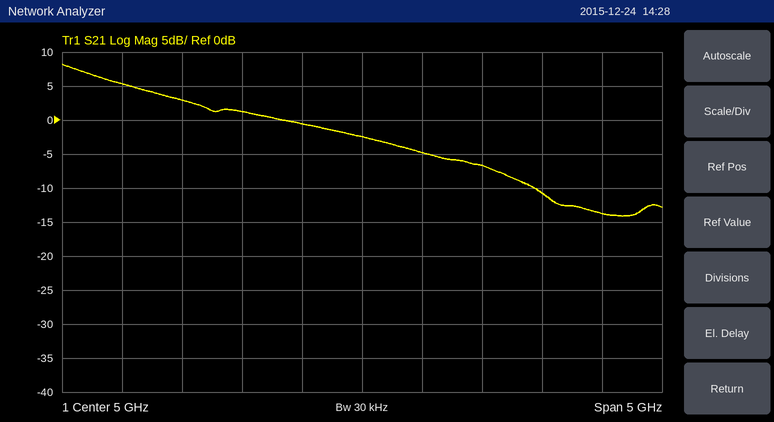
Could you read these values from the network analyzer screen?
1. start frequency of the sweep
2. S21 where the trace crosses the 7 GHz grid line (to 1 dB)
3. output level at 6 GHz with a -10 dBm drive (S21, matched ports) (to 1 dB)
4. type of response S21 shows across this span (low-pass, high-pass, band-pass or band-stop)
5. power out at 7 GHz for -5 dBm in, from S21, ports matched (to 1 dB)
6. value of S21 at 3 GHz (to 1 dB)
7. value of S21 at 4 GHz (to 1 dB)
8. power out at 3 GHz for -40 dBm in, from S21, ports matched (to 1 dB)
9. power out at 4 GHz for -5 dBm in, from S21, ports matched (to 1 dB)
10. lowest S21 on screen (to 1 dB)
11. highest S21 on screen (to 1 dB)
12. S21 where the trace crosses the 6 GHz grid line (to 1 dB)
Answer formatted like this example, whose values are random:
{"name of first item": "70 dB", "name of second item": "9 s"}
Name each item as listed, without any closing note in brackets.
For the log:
{"start frequency of the sweep": "2.5 GHz", "S21 where the trace crosses the 7 GHz grid line": "-14 dB", "output level at 6 GHz with a -10 dBm drive (S21, matched ports)": "-17 dBm", "type of response S21 shows across this span": "low-pass", "power out at 7 GHz for -5 dBm in, from S21, ports matched": "-19 dBm", "value of S21 at 3 GHz": "5 dB", "value of S21 at 4 GHz": "1 dB", "power out at 3 GHz for -40 dBm in, from S21, ports matched": "-35 dBm", "power out at 4 GHz for -5 dBm in, from S21, ports matched": "-4 dBm", "lowest S21 on screen": "-14 dB", "highest S21 on screen": "8 dB", "S21 where the trace crosses the 6 GHz grid line": "-7 dB"}
